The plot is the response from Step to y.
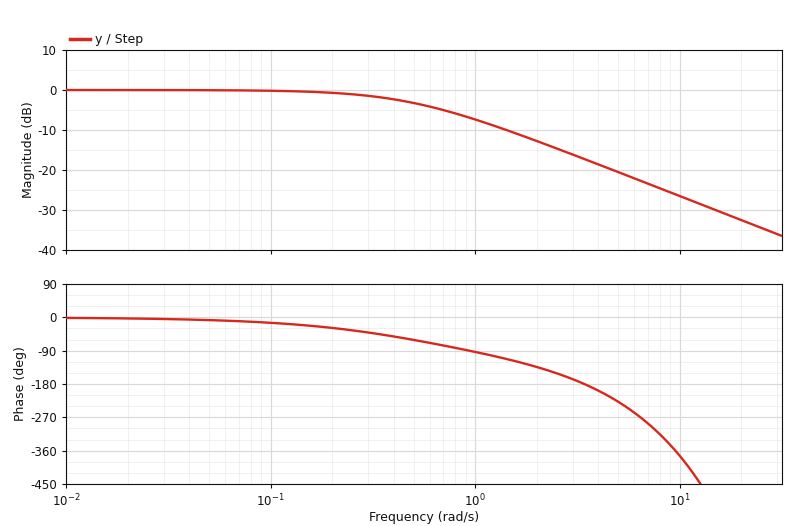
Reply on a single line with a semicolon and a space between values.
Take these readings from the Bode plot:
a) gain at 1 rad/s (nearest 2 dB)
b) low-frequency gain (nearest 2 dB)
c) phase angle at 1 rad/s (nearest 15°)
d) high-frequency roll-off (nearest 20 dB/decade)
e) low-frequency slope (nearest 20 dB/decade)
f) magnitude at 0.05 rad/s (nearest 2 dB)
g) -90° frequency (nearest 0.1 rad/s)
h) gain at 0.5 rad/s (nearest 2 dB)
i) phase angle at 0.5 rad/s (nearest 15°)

-8 dB; 0 dB; -90°; -20 dB/decade; 0 dB/decade; 0 dB; 0.9 rad/s; -4 dB; -60°
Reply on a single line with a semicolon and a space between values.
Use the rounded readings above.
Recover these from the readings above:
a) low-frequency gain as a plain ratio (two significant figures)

1.0
